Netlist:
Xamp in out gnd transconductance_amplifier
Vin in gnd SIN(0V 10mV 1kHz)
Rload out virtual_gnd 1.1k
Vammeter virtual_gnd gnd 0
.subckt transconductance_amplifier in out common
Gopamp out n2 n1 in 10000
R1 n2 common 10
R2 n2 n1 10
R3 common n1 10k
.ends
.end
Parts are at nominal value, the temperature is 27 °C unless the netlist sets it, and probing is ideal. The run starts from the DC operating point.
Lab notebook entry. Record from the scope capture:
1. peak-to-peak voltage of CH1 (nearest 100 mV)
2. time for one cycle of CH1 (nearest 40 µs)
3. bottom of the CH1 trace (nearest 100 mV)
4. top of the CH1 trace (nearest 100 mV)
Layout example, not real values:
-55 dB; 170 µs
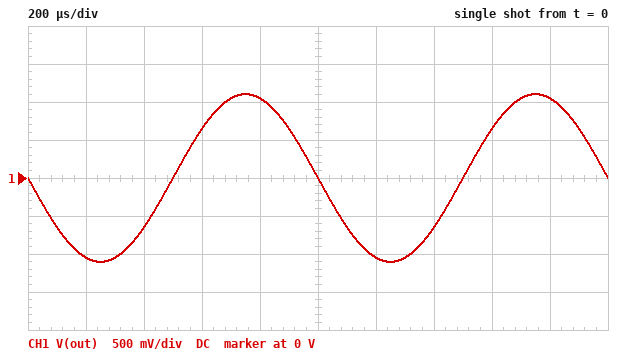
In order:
2.2 V; 1.00 ms; -1.1 V; 1.1 V
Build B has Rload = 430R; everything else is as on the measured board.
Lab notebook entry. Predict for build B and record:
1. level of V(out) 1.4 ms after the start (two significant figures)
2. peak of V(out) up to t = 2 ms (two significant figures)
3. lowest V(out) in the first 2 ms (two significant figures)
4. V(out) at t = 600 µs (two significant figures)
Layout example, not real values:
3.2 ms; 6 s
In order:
-250 mV; 430 mV; -430 mV; 250 mV
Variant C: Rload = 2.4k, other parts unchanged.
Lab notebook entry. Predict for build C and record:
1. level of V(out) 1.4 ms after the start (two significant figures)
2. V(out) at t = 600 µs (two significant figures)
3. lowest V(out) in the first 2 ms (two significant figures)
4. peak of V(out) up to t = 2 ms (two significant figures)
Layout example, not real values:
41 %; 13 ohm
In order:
-1.4 V; 1.4 V; -2.4 V; 2.4 V
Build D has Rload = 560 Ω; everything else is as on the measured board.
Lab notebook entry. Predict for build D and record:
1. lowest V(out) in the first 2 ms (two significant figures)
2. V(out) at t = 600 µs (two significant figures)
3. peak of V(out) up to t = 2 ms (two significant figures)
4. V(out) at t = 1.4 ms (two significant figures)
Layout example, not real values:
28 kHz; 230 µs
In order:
-560 mV; 330 mV; 560 mV; -330 mV
